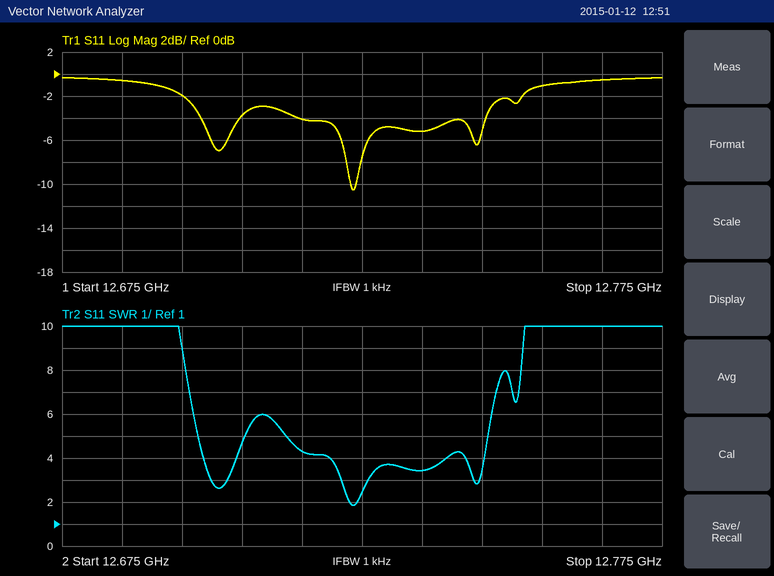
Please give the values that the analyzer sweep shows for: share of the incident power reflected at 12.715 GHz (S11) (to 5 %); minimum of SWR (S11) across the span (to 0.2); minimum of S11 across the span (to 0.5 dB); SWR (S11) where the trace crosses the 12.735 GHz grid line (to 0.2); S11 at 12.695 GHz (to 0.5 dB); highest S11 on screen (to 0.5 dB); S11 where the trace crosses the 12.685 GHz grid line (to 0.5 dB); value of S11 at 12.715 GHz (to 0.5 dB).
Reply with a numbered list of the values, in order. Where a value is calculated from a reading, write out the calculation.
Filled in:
1. 10^(-4/10) ≈ 40 %
2. 1.8
3. -10.5 dB
4. 3.4
5. -2.0 dB
6. -0.5 dB
7. -0.5 dB
8. -4.0 dB
